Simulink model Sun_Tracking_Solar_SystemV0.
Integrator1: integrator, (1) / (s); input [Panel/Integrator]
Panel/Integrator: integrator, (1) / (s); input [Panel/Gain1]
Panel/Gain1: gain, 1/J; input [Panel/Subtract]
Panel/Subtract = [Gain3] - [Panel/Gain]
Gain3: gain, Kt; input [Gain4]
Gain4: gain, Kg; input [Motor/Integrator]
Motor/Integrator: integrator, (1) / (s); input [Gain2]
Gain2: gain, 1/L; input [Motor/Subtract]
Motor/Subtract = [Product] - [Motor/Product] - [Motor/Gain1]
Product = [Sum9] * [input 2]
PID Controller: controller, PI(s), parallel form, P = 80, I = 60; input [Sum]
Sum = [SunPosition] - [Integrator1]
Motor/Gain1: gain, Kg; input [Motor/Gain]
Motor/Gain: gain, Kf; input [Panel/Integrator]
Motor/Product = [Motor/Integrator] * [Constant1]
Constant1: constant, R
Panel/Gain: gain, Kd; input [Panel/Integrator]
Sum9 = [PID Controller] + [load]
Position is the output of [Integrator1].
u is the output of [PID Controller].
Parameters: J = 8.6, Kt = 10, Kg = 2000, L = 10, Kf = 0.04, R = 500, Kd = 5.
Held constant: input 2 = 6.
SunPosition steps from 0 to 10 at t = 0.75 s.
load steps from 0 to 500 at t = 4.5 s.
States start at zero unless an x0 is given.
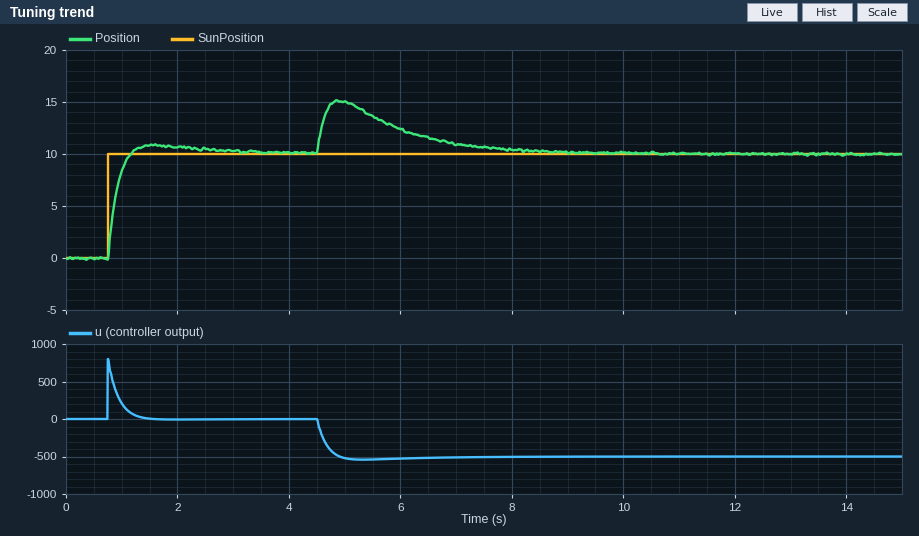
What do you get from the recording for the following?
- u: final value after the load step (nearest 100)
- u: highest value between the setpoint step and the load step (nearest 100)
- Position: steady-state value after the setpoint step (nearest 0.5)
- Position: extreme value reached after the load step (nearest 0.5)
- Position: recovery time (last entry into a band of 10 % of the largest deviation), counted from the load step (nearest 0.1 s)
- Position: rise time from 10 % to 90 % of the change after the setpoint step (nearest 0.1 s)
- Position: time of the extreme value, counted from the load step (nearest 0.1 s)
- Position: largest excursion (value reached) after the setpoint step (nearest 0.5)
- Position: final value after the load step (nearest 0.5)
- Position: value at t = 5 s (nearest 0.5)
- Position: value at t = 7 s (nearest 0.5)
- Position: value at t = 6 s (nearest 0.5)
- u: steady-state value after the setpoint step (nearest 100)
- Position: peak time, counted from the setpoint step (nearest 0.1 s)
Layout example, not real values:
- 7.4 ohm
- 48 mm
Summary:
- -500
- 800
- 10.0
- 15.0
- 3.3 s
- 0.3 s
- 0.4 s
- 11.0
- 10.0
- 15.0
- 11.0
- 12.5
- 0
- 0.8 s
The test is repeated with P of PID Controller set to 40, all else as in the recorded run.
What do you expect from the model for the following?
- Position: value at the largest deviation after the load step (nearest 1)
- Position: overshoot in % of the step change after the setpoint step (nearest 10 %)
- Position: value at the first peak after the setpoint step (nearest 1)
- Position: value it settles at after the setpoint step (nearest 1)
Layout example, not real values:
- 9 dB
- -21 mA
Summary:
- 18
- 20 %
- 12
- 10
